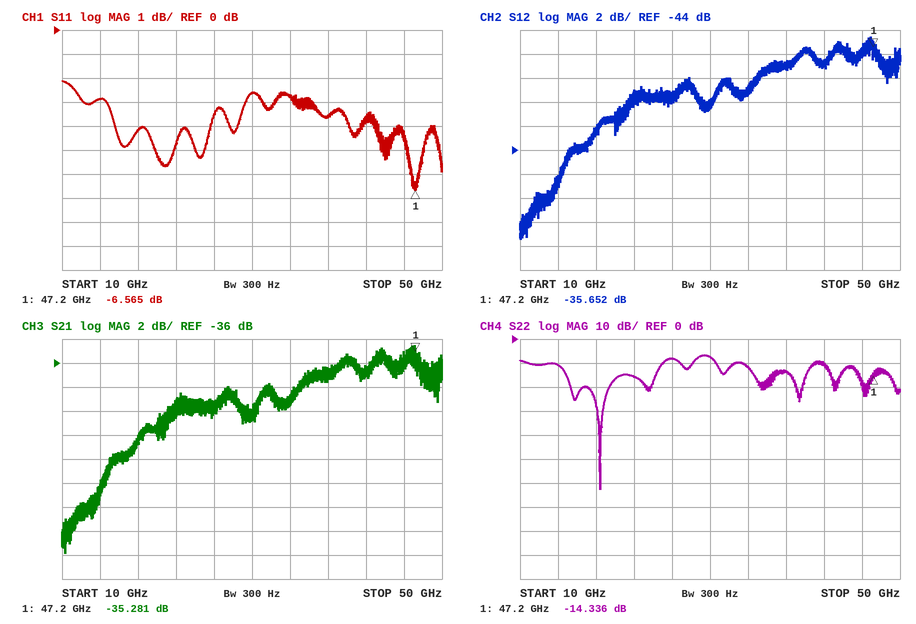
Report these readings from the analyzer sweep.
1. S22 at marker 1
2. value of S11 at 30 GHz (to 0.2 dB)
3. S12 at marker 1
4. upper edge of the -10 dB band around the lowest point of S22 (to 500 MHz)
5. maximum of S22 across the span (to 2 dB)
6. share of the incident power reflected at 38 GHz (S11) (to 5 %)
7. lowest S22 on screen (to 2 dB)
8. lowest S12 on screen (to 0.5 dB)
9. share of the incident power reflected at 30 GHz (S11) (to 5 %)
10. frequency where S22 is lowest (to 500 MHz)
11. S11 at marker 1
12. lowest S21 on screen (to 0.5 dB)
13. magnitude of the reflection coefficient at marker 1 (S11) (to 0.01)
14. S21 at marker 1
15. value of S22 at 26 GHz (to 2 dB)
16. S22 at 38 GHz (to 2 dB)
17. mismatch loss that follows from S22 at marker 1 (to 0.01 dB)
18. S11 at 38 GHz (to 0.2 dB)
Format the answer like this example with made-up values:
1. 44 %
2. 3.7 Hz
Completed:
1. -14.336 dB
2. -2.6 dB
3. -35.652 dB
4. 25.0 GHz
5. -6 dB
6. 45 %
7. -62 dB
8. -51.5 dB
9. 55 %
10. 18.5 GHz
11. -6.565 dB
12. -52.0 dB
13. 0.47
14. -35.281 dB
15. -8 dB
16. -14 dB
17. 0.16 dB
18. -3.6 dB
